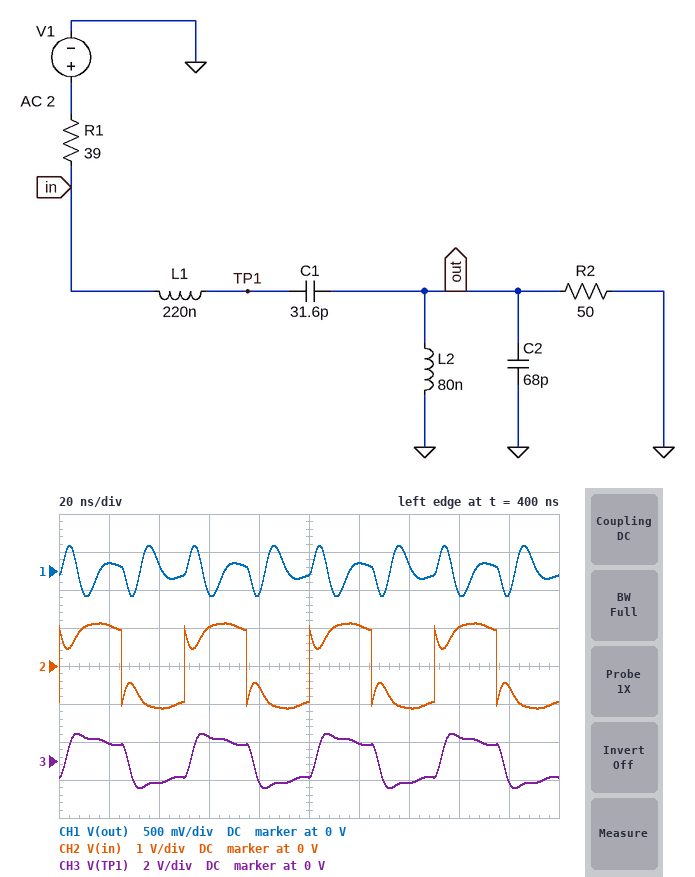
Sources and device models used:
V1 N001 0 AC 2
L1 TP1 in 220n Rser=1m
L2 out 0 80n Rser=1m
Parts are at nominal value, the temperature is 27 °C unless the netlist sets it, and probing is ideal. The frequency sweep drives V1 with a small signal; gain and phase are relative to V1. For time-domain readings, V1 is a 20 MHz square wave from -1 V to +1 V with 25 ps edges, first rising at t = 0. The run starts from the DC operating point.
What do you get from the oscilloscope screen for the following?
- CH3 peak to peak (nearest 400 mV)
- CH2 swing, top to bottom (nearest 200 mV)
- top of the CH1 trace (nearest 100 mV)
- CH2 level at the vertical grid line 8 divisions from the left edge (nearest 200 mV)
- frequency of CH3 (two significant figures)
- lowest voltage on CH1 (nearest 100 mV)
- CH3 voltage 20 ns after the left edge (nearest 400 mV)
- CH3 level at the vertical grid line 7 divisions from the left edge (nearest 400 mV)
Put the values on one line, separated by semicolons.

2.8 V; 2.2 V; 300 mV; 1.0 V; 20 MHz; -300 mV; 800 mV; -1.2 V
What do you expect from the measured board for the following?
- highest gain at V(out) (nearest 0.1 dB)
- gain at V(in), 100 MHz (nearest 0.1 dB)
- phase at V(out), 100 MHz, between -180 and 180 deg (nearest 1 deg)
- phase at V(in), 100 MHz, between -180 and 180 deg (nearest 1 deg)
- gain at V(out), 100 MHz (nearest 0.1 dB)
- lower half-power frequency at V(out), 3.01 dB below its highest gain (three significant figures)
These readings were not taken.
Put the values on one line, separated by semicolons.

-5.0 dB; -2.4 dB; -95 deg; 25 deg; -8.5 dB; 41.2 MHz
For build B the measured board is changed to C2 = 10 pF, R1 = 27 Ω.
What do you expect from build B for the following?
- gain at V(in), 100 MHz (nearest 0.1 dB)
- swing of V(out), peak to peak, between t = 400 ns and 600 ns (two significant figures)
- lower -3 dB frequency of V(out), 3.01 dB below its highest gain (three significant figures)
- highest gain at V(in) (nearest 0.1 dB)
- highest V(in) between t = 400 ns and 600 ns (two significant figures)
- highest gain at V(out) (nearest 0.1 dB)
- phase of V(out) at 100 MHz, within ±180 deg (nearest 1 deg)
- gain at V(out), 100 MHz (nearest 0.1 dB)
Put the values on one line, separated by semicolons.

-0.8 dB; 840 mV; 44.7 MHz; 0 dB; 1.2 V; -3.9 dB; -27 deg; -9.7 dB
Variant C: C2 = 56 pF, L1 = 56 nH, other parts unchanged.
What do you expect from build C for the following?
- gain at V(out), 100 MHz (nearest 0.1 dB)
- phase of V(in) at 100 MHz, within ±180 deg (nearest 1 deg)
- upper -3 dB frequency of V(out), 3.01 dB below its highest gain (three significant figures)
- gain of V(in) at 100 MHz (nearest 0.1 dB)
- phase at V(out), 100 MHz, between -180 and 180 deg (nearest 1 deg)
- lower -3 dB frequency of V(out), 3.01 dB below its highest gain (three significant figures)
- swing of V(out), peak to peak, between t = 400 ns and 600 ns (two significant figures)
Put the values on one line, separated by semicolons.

-6.2 dB; -22 deg; 180 MHz; -4.1 dB; -8 deg; 48.0 MHz; 1.0 V
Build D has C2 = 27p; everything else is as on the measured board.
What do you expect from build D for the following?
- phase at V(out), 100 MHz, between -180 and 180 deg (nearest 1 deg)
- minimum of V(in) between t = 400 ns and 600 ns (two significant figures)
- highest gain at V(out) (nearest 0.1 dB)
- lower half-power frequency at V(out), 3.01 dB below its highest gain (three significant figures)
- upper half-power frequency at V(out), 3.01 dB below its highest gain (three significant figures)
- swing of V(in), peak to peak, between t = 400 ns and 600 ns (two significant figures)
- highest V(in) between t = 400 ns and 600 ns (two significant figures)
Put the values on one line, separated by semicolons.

-39 deg; -1.2 V; -5.7 dB; 43.0 MHz; 108 MHz; 2.4 V; 1.2 V
